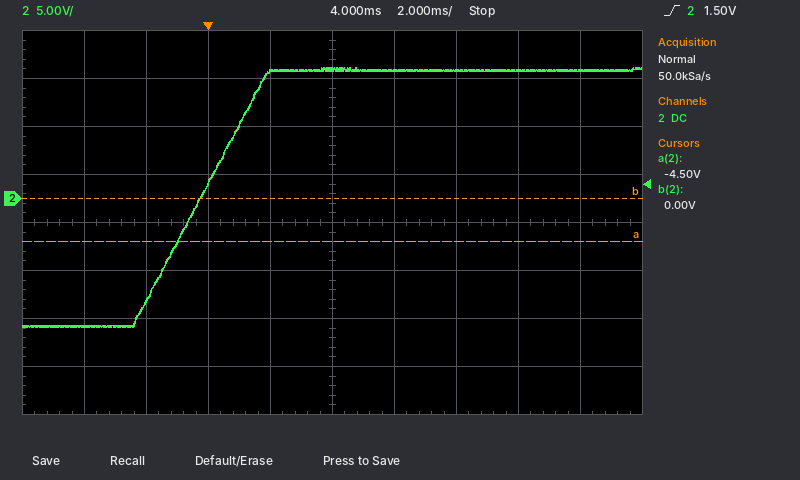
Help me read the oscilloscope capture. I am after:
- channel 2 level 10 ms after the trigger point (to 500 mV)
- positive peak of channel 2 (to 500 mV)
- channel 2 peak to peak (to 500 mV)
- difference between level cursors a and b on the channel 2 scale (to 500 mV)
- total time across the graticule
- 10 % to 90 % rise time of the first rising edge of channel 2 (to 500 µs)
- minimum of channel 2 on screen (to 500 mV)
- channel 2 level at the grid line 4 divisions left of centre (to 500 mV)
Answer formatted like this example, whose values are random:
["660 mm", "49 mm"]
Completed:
["13.5 V", "13.5 V", "27.0 V", "4.5 V", "20 ms", "3.5 ms", "-13.5 V", "-13.5 V"]
